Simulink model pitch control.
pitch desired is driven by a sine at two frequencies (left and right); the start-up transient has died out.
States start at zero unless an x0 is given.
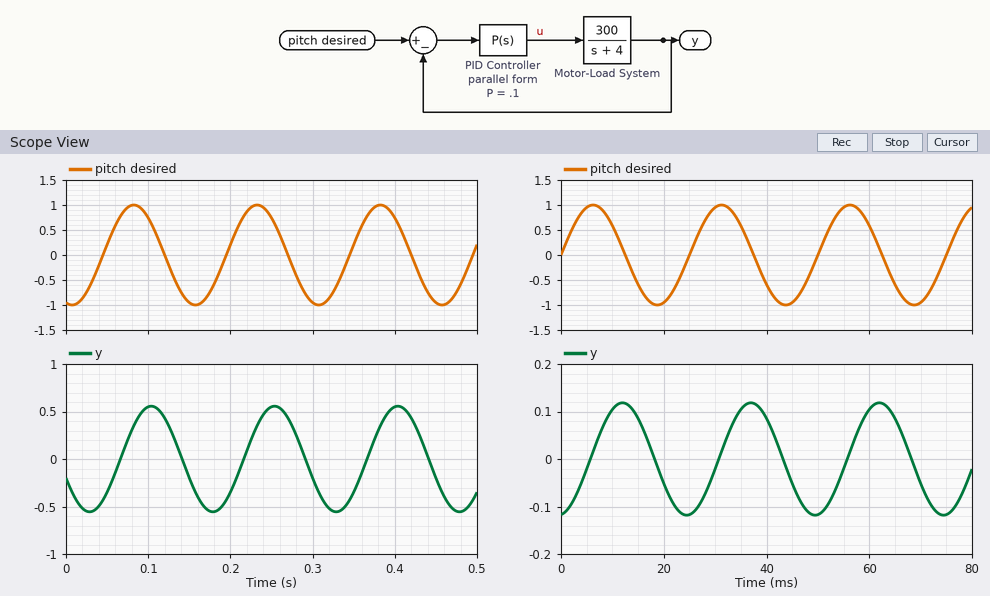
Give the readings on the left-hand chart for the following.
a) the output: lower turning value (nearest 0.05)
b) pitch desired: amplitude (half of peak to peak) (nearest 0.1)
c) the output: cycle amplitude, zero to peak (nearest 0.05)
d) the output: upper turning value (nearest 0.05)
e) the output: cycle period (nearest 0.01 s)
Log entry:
-0.55
1.0
0.55
0.55
0.15 s
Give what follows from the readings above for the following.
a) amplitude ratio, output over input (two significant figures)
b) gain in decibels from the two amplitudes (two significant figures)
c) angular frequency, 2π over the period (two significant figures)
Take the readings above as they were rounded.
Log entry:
0.55
-5.2 dB
42 rad/s
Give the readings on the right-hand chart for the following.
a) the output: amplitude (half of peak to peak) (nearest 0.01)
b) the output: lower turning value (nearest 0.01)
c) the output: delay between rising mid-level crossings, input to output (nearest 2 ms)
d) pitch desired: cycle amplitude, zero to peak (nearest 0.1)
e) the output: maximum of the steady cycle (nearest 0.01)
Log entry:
0.12
-0.12
6 ms
1.0
0.12
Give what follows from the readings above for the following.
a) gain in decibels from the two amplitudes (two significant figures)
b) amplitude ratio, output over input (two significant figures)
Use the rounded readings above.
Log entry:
-18 dB
0.12
